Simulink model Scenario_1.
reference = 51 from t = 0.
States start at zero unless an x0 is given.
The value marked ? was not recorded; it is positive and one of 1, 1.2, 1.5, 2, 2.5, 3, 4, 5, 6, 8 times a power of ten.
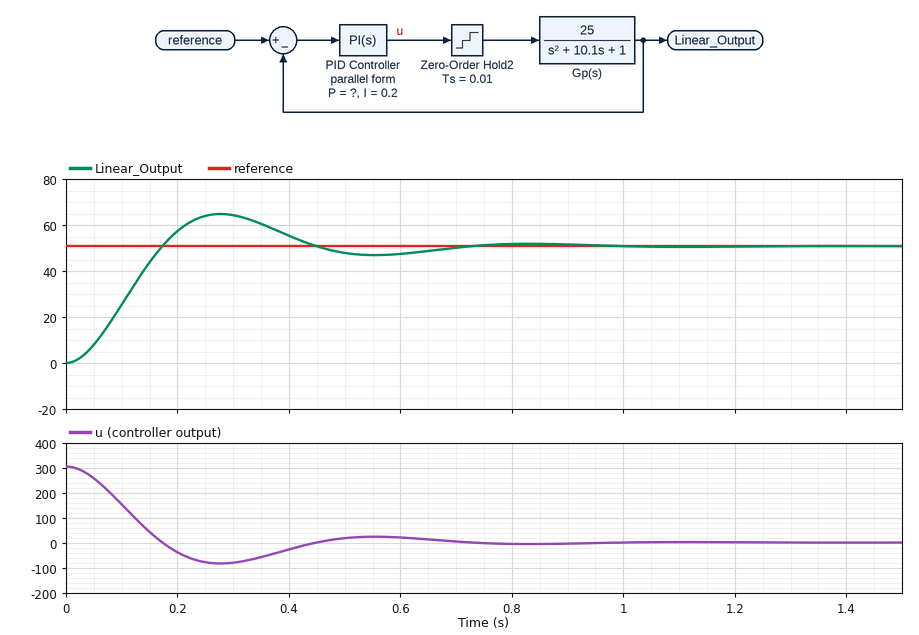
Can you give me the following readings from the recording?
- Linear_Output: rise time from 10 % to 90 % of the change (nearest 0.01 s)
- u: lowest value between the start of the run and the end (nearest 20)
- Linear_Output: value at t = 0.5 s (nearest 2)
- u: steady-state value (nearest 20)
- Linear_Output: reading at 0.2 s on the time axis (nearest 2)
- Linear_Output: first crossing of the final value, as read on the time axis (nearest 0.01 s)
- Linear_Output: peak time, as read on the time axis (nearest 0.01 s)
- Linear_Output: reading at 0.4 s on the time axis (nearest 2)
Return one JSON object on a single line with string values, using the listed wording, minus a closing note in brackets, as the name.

{"Linear_Output: rise time from 10 % to 90 % of the change": "0.12 s", "u: lowest value between the start of the run and the end": "-80", "Linear_Output: value at t = 0.5 s": "48", "u: steady-state value": "0", "Linear_Output: reading at 0.2 s on the time axis": "58", "Linear_Output: first crossing of the final value, as read on the time axis": "0.17 s", "Linear_Output: peak time, as read on the time axis": "0.28 s", "Linear_Output: reading at 0.4 s on the time axis": "56"}
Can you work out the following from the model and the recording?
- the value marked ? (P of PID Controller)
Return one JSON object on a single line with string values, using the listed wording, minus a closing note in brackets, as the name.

{"the value marked ?": "6"}
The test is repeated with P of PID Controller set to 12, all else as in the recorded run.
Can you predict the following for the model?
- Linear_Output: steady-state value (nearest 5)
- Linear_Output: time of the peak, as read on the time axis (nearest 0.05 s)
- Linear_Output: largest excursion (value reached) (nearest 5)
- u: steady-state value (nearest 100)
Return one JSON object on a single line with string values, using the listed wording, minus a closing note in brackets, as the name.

{"Linear_Output: steady-state value": "50", "Linear_Output: time of the peak, as read on the time axis": "0.20 s", "Linear_Output: largest excursion (value reached)": "75", "u: steady-state value": "0"}
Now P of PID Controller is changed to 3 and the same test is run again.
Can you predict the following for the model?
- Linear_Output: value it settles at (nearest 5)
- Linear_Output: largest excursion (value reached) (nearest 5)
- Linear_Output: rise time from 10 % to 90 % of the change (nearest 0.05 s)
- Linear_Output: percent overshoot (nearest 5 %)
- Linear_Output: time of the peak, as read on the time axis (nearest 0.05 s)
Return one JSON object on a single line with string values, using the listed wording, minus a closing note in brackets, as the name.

{"Linear_Output: value it settles at": "50", "Linear_Output: largest excursion (value reached)": "55", "Linear_Output: rise time from 10 % to 90 % of the change": "0.20 s", "Linear_Output: percent overshoot": "10 %", "Linear_Output: time of the peak, as read on the time axis": "0.45 s"}
